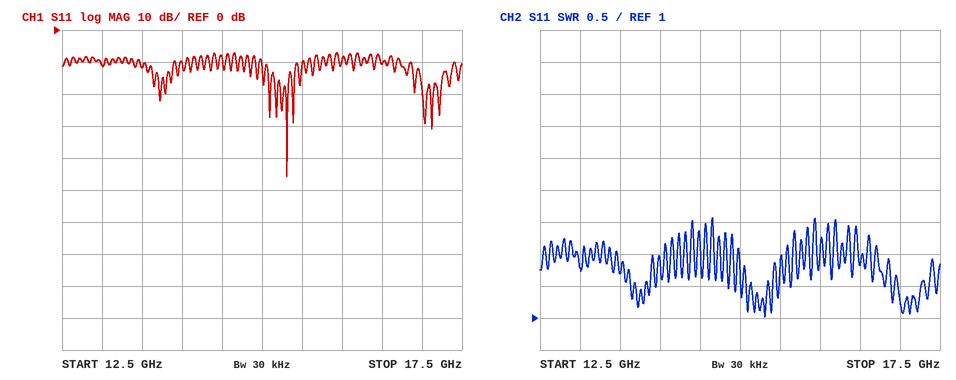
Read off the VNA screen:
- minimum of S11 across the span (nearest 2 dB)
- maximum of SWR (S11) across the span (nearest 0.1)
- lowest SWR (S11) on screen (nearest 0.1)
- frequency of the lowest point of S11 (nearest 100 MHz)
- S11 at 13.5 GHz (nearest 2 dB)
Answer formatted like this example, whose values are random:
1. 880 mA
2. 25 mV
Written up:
1. -46 dB
2. 2.6
3. 1.0
4. 15.3 GHz
5. -12 dB
